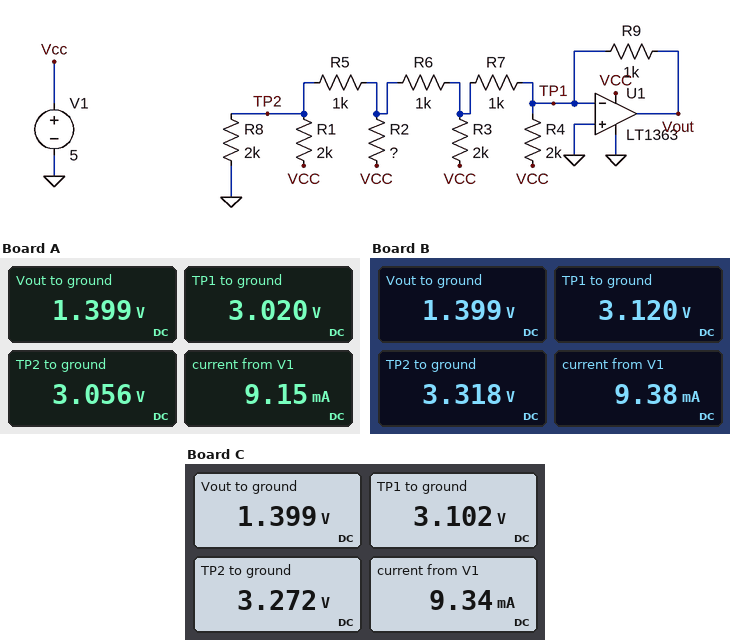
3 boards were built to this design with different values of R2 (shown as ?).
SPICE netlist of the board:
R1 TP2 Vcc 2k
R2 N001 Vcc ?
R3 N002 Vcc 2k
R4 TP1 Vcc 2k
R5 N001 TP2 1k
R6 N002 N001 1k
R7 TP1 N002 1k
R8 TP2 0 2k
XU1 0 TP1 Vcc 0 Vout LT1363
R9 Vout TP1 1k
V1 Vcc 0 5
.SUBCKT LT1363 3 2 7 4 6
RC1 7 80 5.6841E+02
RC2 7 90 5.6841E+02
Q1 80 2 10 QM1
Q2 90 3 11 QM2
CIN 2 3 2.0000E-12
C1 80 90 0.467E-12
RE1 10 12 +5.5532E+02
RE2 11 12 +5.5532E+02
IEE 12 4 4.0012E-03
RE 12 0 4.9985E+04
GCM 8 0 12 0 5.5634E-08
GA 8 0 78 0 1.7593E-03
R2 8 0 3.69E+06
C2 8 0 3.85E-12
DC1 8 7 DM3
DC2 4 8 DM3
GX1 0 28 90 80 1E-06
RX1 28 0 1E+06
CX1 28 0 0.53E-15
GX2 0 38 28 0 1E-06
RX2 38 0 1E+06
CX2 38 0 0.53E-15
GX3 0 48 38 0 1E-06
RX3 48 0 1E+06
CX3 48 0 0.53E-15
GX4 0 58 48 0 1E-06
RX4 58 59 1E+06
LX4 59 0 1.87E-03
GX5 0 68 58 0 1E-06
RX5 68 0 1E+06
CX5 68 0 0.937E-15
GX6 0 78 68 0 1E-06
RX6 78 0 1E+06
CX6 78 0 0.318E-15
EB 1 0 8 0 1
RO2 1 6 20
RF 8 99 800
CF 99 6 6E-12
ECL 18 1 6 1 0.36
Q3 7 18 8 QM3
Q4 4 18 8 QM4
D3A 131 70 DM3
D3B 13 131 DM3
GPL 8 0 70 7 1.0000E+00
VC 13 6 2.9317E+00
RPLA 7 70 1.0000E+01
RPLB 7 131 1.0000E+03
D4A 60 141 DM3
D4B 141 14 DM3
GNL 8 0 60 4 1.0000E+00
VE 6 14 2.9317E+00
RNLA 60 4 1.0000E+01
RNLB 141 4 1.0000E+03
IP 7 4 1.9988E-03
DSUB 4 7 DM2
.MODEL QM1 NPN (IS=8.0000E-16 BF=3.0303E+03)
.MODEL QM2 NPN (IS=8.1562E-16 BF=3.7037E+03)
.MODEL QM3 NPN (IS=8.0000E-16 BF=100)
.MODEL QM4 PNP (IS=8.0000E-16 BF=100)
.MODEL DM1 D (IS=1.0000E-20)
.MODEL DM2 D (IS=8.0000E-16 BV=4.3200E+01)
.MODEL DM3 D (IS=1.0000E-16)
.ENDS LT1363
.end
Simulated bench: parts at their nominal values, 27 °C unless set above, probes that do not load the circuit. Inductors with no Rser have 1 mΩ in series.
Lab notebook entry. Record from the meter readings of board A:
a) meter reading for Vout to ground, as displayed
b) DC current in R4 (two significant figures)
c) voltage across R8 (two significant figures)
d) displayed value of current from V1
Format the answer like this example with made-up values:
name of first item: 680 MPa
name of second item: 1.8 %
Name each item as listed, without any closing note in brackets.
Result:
meter reading for Vout to ground, as displayed: 1.399 V
DC current in R4: 990 µA
voltage across R8: 3.1 V
displayed value of current from V1: 9.15 mA
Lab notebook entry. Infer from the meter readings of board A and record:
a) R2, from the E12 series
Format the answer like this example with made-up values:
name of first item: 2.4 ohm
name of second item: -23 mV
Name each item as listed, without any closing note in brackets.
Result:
R2, from the E12 series: 2.7 kΩ
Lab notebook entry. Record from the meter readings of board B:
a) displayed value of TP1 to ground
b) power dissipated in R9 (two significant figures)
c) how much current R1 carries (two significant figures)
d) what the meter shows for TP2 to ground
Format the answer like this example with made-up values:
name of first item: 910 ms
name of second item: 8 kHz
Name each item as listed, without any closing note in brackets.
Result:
displayed value of TP1 to ground: 3.120 V
power dissipated in R9: 3.0 mW
how much current R1 carries: 840 µA
what the meter shows for TP2 to ground: 3.318 V
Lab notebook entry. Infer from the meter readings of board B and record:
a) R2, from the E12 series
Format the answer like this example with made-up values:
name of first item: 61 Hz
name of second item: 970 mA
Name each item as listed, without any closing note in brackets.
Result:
R2, from the E12 series: 820 Ω
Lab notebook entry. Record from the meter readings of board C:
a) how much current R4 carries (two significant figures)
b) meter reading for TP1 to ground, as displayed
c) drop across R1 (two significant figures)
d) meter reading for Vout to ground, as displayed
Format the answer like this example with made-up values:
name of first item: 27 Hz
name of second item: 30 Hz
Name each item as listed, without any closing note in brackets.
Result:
how much current R4 carries: 950 µA
meter reading for TP1 to ground, as displayed: 3.102 V
drop across R1: 1.7 V
meter reading for Vout to ground, as displayed: 1.399 V
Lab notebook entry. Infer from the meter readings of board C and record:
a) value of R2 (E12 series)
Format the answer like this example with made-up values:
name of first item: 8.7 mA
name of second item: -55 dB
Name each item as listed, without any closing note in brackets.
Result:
value of R2: 1 kΩ
